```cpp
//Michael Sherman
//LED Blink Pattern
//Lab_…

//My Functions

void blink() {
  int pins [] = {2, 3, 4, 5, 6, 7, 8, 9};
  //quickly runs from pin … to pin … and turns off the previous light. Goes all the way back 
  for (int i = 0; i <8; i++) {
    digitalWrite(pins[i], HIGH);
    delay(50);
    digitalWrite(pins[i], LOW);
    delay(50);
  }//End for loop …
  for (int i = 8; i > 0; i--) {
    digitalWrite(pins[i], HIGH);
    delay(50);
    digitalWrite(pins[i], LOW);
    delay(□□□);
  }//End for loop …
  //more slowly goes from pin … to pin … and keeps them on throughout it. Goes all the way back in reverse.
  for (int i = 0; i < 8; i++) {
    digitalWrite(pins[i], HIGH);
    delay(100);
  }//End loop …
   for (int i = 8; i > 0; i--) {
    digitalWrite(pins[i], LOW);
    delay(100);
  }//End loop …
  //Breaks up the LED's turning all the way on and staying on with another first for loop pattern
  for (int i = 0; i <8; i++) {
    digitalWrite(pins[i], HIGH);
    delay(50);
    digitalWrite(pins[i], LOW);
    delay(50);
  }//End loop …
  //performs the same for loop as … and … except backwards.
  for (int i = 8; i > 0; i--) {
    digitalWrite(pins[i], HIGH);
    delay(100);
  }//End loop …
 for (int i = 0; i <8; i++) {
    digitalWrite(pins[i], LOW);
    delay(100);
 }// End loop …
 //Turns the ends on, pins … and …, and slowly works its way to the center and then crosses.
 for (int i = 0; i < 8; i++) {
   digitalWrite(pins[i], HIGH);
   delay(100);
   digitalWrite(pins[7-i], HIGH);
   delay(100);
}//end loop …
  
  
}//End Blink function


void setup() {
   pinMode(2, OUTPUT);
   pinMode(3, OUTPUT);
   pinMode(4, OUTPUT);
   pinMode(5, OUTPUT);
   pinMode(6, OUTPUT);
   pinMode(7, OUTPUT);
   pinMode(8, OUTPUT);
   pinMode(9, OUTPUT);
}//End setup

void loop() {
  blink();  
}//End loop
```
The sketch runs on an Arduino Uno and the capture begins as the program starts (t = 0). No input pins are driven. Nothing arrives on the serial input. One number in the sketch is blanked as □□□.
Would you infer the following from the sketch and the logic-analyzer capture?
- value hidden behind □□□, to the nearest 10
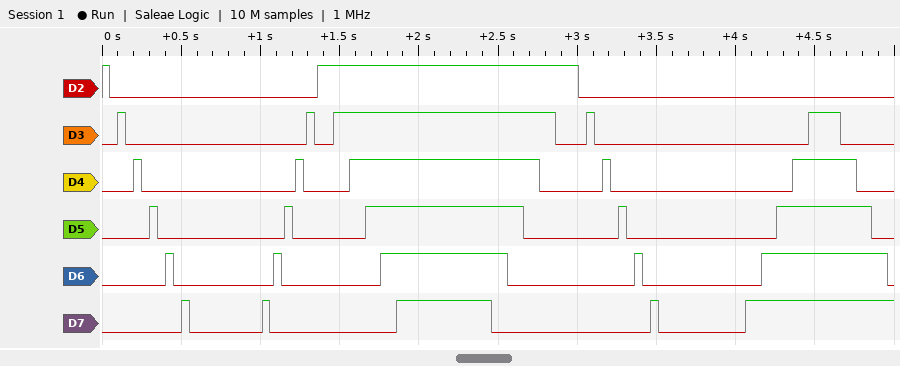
20
